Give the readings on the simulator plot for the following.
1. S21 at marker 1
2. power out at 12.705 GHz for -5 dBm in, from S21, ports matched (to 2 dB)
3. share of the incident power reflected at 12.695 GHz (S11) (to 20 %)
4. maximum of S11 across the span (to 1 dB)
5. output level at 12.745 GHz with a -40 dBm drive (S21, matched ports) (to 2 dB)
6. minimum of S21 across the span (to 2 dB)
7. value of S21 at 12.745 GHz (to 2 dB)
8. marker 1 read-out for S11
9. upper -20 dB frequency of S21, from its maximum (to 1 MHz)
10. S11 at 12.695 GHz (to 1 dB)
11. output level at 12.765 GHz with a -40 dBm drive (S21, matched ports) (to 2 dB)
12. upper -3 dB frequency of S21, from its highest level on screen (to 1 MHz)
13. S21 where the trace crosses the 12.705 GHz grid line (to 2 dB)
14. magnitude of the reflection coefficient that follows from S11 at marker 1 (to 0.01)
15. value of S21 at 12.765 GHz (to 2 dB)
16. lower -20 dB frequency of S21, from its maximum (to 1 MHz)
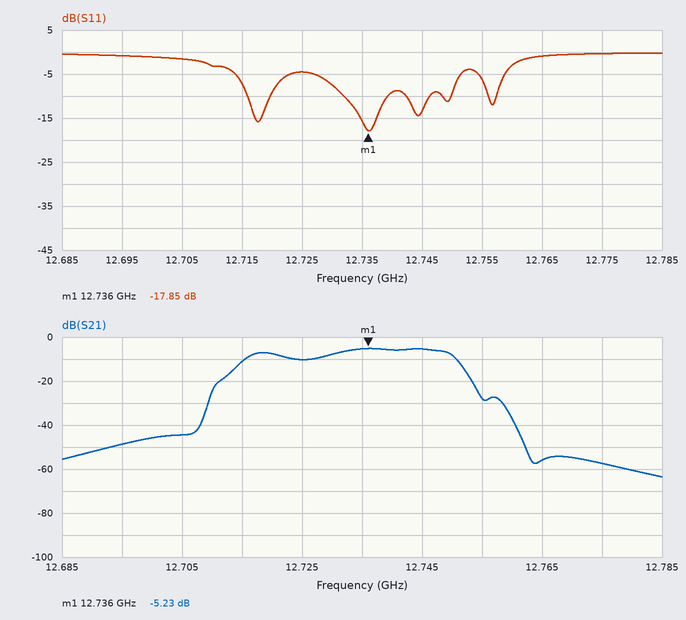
-5.23 dB
-50 dBm
80 %
0 dB
-46 dBm
-64 dB
-6 dB
-17.85 dB
12.754 GHz
-1 dB
-96 dBm
12.750 GHz
-44 dB
0.13
-56 dB
12.710 GHz
